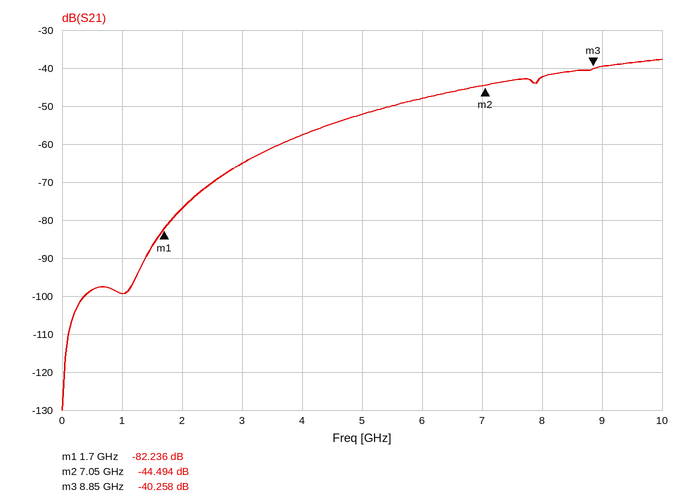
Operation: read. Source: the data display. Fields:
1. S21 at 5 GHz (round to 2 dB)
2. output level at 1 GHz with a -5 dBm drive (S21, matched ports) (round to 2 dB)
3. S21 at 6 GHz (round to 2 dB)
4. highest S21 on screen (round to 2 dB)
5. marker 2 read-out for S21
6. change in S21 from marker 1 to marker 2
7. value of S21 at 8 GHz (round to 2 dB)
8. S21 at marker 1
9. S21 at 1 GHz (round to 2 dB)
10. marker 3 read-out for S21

-52 dB
-104 dBm
-48 dB
-38 dB
-44.494 dB
37.742 dB
-42 dB
-82.236 dB
-100 dB
-40.258 dB
